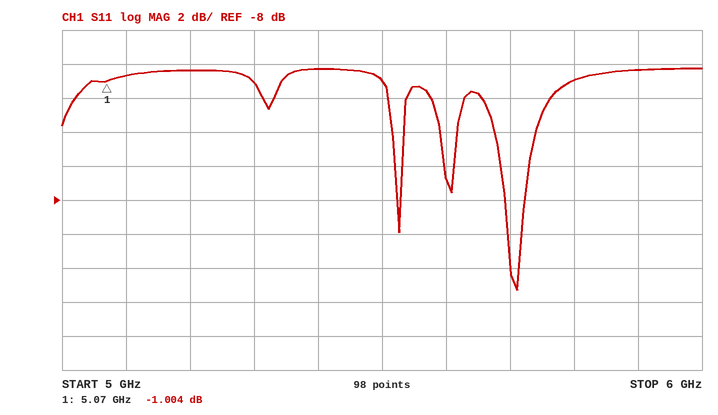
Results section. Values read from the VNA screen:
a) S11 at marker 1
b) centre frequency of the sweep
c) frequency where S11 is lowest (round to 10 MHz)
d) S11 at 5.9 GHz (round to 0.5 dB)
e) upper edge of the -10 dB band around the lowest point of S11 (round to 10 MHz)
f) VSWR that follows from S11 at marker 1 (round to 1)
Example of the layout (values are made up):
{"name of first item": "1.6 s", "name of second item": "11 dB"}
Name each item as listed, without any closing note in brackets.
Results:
{"S11 at marker 1": "-1.004 dB", "centre frequency of the sweep": "5.5 GHz", "frequency where S11 is lowest": "5.71 GHz", "S11 at 5.9 GHz": "-0.5 dB", "upper edge of the -10 dB band around the lowest point of S11": "5.72 GHz", "VSWR that follows from S11 at marker 1": "17"}
